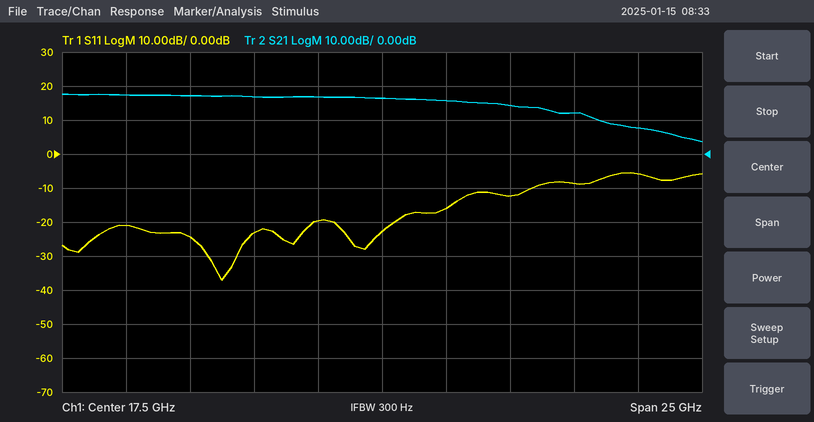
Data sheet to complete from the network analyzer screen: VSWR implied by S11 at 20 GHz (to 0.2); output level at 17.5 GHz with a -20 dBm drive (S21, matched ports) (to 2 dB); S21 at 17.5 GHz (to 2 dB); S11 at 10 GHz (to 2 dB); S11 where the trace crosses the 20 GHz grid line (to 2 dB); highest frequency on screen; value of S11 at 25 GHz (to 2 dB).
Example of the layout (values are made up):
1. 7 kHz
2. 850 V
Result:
1. 1.4
2. -4 dBm
3. 16 dB
4. -24 dB
5. -16 dB
6. 30 GHz
7. -8 dB
